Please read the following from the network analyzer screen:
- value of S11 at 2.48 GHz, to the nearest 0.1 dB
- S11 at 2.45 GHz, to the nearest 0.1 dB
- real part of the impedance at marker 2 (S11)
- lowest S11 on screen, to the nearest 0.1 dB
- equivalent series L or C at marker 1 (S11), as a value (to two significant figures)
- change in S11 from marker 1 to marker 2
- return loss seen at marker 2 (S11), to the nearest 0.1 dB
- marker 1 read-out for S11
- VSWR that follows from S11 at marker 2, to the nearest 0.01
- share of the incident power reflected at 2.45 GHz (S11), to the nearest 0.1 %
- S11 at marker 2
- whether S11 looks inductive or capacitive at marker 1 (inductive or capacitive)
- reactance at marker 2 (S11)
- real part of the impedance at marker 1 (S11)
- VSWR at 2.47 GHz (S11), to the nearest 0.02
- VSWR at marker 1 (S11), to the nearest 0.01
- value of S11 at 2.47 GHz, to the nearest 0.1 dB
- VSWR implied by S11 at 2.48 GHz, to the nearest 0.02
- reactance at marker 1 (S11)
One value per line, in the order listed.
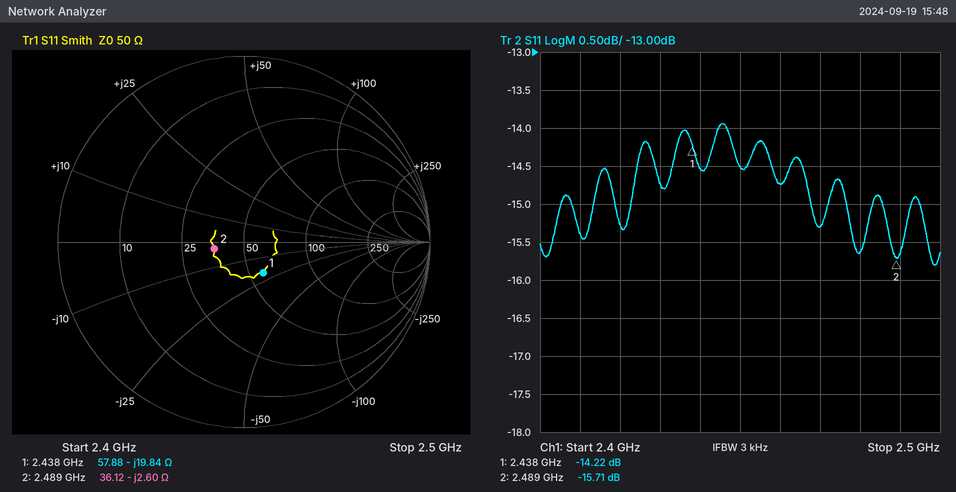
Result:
-15.6 dB
-14.5 dB
36.12 Ω
-15.8 dB
3.3 pF
-1.49 dB
15.7 dB
-14.22 dB
1.39
3.5 %
-15.71 dB
capacitive
-2.60 Ω
57.88 Ω
1.42
1.48
-15.3 dB
1.40
-19.84 Ω
